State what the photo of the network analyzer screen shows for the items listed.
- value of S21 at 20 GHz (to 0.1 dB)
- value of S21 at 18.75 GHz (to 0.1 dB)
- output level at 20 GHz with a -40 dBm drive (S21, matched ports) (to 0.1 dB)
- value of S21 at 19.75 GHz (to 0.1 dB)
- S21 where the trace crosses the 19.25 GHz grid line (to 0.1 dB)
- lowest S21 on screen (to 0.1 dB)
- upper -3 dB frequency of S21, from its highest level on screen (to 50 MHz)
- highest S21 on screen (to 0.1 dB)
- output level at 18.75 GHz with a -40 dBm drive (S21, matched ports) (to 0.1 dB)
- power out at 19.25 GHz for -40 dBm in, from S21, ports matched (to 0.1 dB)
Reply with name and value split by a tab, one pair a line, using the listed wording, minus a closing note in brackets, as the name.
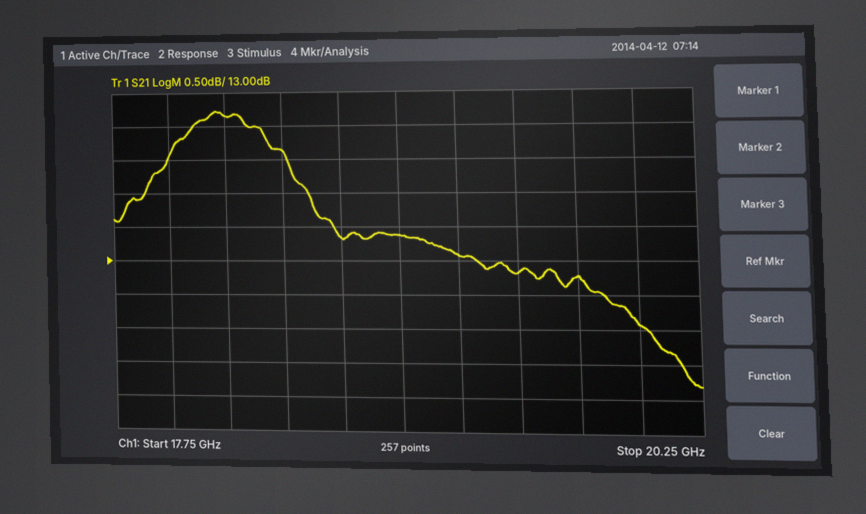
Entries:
value of S21 at 20 GHz	12.1 dB
value of S21 at 18.75 GHz	13.3 dB
output level at 20 GHz with a -40 dBm drive (S21, matched ports)	-27.9 dBm
value of S21 at 19.75 GHz	12.8 dB
S21 where the trace crosses the 19.25 GHz grid line	13.1 dB
lowest S21 on screen	11.2 dB
upper -3 dB frequency of S21, from its highest level on screen	19.95 GHz
highest S21 on screen	15.2 dB
output level at 18.75 GHz with a -40 dBm drive (S21, matched ports)	-26.7 dBm
power out at 19.25 GHz for -40 dBm in, from S21, ports matched	-26.9 dBm
